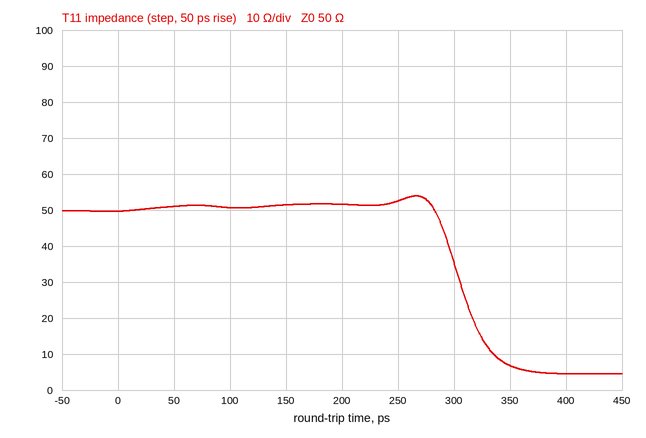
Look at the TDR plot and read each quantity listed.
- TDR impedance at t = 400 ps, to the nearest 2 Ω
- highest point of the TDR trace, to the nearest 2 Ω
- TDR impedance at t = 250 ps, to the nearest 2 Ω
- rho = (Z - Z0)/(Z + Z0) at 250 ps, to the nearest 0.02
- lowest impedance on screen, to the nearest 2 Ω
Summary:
4 Ω
54 Ω
52 Ω
+0.02
4 Ω
